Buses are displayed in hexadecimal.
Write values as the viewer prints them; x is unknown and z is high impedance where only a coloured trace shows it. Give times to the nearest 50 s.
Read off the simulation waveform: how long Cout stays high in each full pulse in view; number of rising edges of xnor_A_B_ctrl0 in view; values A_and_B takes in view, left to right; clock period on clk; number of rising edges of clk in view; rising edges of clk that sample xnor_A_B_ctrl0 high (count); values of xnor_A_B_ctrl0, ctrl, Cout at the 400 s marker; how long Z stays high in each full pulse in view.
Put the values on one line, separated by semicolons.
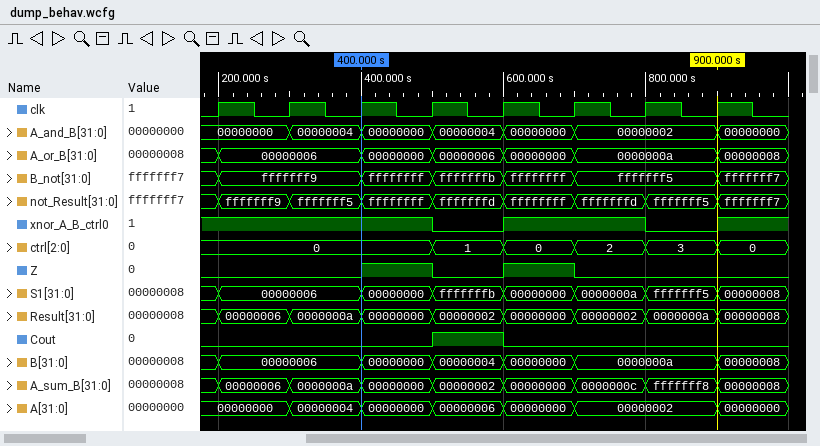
100 s; 2; 00000000, 00000004, 00000000, 00000004, 00000000, 00000002, 00000000; 100 s; 8; 6; xnor_A_B_ctrl0=1, ctrl=0, Cout=0; 100 s, 100 s
